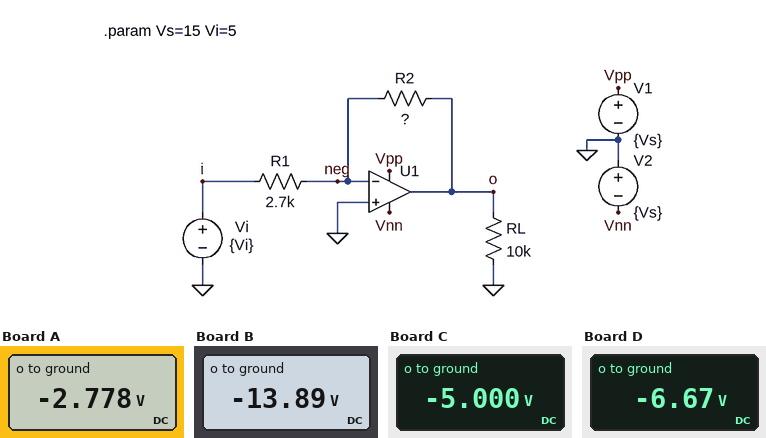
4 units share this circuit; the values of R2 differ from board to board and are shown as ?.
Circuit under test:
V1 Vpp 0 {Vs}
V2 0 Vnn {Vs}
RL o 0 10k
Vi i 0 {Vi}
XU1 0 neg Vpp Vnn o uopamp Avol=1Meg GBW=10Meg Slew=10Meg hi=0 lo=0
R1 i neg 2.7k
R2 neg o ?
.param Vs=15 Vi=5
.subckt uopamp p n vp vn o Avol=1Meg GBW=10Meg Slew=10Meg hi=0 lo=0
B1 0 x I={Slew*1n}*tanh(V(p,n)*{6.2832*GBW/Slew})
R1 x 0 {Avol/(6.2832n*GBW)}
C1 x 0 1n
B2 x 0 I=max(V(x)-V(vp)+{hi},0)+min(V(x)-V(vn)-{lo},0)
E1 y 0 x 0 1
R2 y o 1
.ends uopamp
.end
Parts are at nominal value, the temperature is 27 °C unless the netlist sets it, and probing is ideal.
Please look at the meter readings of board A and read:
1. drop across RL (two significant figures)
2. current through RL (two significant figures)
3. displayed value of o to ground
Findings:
2.8 V
280 µA
-2.778 V
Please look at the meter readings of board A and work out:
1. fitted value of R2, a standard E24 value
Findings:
1.5 kΩ
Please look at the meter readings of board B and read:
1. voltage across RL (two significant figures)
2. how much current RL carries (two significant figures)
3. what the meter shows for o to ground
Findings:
14 V
1.4 mA
-13.89 V
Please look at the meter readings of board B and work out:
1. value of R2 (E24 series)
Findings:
7.5 kΩ
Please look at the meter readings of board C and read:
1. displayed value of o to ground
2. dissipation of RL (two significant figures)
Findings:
-5.000 V
2.5 mW
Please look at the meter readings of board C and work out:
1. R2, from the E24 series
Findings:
2.7 kΩ
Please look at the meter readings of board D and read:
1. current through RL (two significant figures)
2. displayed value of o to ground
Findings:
670 µA
-6.67 V
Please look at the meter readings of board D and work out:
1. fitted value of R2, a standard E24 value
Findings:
3.6 kΩ
